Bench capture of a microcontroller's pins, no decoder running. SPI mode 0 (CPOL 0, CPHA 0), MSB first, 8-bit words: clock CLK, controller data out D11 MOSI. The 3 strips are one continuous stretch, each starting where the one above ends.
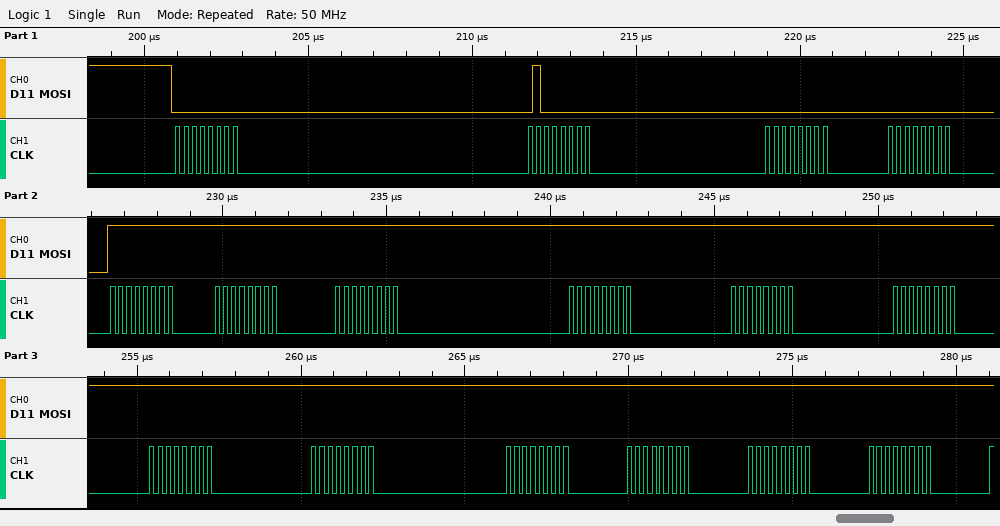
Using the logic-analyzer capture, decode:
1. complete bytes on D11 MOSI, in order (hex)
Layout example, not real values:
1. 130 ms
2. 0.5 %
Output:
1. 00 40 00 00 FF FF FF FF FF FF FF FF FF FF FF FF
